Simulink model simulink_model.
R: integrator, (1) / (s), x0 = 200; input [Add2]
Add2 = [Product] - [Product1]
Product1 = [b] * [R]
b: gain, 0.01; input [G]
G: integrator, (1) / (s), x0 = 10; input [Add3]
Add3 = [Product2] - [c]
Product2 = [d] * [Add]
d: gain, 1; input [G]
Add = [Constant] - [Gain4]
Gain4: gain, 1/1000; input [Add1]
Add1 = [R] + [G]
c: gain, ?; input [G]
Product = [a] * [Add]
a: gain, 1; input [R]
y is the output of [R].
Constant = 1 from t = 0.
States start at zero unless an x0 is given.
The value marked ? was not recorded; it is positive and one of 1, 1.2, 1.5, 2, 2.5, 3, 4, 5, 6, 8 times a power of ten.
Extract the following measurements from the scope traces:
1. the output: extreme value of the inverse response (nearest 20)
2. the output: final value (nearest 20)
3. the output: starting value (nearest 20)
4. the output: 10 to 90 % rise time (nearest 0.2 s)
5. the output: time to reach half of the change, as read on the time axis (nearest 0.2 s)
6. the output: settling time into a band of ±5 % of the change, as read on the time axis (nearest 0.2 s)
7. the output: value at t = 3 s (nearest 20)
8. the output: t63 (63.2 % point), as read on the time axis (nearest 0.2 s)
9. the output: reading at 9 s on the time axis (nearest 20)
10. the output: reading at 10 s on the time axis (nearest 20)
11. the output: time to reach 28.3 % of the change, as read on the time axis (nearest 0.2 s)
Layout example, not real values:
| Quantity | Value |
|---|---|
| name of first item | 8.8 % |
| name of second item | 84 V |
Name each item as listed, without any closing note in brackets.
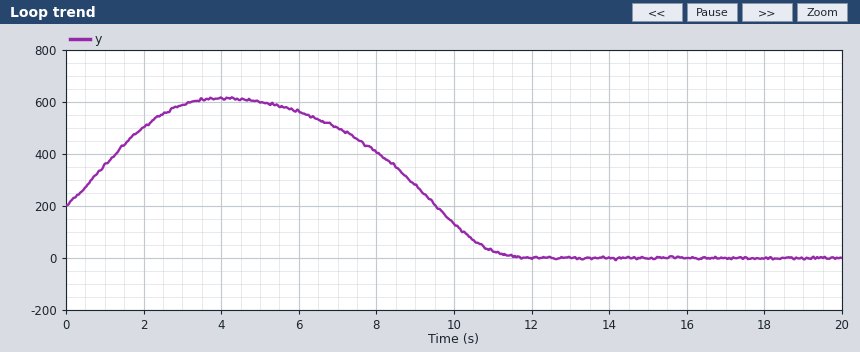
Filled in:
| Quantity | Value |
|---|---|
| the output: extreme value of the inverse response | 620 |
| the output: final value | 0 |
| the output: starting value | 200 |
| the output: 10 to 90 % rise time | 1.4 s |
| the output: time to reach half of the change, as read on the time axis | 10.2 s |
| the output: settling time into a band of ±5 % of the change, as read on the time axis | 11.4 s |
| the output: value at t = 3 s | 580 |
| the output: t63 (63.2 % point), as read on the time axis | 10.4 s |
| the output: reading at 9 s on the time axis | 280 |
| the output: reading at 10 s on the time axis | 140 |
| the output: time to reach 28.3 % of the change, as read on the time axis | 10.0 s |
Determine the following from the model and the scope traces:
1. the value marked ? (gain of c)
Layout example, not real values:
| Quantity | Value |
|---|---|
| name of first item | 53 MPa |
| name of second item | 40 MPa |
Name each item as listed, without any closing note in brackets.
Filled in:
| Quantity | Value |
|---|---|
| the value marked ? | 0.2 |
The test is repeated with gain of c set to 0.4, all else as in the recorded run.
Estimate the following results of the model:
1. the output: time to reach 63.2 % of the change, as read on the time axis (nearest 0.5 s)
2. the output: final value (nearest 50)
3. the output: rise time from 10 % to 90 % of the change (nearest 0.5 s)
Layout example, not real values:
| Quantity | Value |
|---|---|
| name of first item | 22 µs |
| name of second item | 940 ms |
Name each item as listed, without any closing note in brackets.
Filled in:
| Quantity | Value |
|---|---|
| the output: time to reach 63.2 % of the change, as read on the time axis | 3.5 s |
| the output: final value | 1000 |
| the output: rise time from 10 % to 90 % of the change | 7.5 s |
